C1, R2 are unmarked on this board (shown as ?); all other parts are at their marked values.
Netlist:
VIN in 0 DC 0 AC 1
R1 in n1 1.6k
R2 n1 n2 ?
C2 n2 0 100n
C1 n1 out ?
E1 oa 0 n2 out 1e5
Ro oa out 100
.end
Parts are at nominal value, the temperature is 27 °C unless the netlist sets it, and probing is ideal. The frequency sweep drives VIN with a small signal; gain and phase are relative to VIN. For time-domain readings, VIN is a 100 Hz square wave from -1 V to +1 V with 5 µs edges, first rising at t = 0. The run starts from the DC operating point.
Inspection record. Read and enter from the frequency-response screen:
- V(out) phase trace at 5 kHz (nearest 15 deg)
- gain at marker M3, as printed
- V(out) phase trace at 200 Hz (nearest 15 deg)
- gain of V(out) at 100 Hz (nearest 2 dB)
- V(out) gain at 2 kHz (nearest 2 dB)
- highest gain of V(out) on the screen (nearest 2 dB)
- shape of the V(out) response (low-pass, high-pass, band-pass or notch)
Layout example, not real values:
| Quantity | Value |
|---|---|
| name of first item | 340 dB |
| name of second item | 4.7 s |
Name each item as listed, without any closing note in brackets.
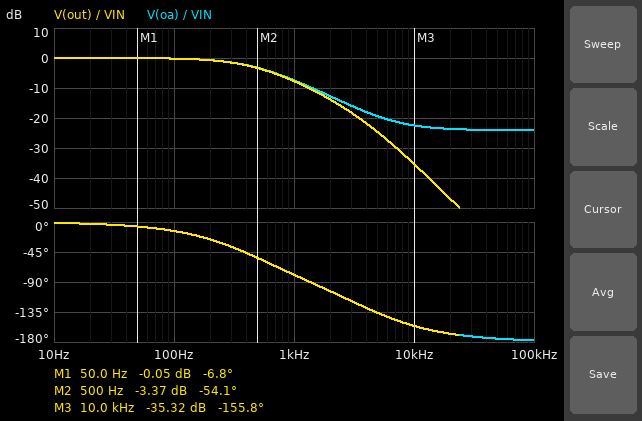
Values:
| Quantity | Value |
|---|---|
| V(out) phase trace at 5 kHz | -135 deg |
| gain at marker M3, as printed | -35.32 dB |
| V(out) phase trace at 200 Hz | -30 deg |
| gain of V(out) at 100 Hz | 0 dB |
| V(out) gain at 2 kHz | -14 dB |
| highest gain of V(out) on the screen | 0 dB |
| shape of the V(out) response | low-pass |
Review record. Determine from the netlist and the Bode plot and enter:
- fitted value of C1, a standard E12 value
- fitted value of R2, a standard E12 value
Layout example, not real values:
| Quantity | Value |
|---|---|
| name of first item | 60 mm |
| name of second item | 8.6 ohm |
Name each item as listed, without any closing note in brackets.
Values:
| Quantity | Value |
|---|---|
| fitted value of C1, a standard E12 value | 39 nF |
| fitted value of R2, a standard E12 value | 2.2 kΩ |
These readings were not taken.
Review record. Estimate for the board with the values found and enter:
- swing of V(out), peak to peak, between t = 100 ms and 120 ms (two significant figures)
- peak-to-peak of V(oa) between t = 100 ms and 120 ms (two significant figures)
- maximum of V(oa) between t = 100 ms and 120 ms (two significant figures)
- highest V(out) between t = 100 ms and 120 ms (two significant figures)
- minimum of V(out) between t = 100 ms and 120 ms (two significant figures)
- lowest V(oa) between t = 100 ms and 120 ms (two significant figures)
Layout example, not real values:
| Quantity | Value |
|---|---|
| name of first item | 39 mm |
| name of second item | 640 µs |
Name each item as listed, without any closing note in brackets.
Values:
| Quantity | Value |
|---|---|
| swing of V(out), peak to peak, between t = 100 ms and 120 ms | 2.0 V |
| peak-to-peak of V(oa) between t = 100 ms and 120 ms | 2.2 V |
| maximum of V(oa) between t = 100 ms and 120 ms | 1.1 V |
| highest V(out) between t = 100 ms and 120 ms | 1.0 V |
| minimum of V(out) between t = 100 ms and 120 ms | -1.0 V |
| lowest V(oa) between t = 100 ms and 120 ms | -1.1 V |
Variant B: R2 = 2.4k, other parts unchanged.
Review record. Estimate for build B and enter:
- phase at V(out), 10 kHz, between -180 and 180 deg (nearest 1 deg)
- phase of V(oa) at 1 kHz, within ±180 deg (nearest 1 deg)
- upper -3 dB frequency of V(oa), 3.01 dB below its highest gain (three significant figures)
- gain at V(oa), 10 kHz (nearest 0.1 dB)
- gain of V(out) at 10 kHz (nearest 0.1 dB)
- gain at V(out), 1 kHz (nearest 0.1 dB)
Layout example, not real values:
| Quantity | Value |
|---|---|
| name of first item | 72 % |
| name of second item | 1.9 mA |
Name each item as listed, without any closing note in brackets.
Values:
| Quantity | Value |
|---|---|
| phase at V(out), 10 kHz, between -180 and 180 deg | -157 deg |
| phase of V(oa) at 1 kHz, within ±180 deg | -81 deg |
| upper -3 dB frequency of V(oa), 3.01 dB below its highest gain | 445 Hz |
| gain at V(oa), 10 kHz | -22.6 dB |
| gain of V(out) at 10 kHz | -36.0 dB |
| gain at V(out), 1 kHz | -8.1 dB |
